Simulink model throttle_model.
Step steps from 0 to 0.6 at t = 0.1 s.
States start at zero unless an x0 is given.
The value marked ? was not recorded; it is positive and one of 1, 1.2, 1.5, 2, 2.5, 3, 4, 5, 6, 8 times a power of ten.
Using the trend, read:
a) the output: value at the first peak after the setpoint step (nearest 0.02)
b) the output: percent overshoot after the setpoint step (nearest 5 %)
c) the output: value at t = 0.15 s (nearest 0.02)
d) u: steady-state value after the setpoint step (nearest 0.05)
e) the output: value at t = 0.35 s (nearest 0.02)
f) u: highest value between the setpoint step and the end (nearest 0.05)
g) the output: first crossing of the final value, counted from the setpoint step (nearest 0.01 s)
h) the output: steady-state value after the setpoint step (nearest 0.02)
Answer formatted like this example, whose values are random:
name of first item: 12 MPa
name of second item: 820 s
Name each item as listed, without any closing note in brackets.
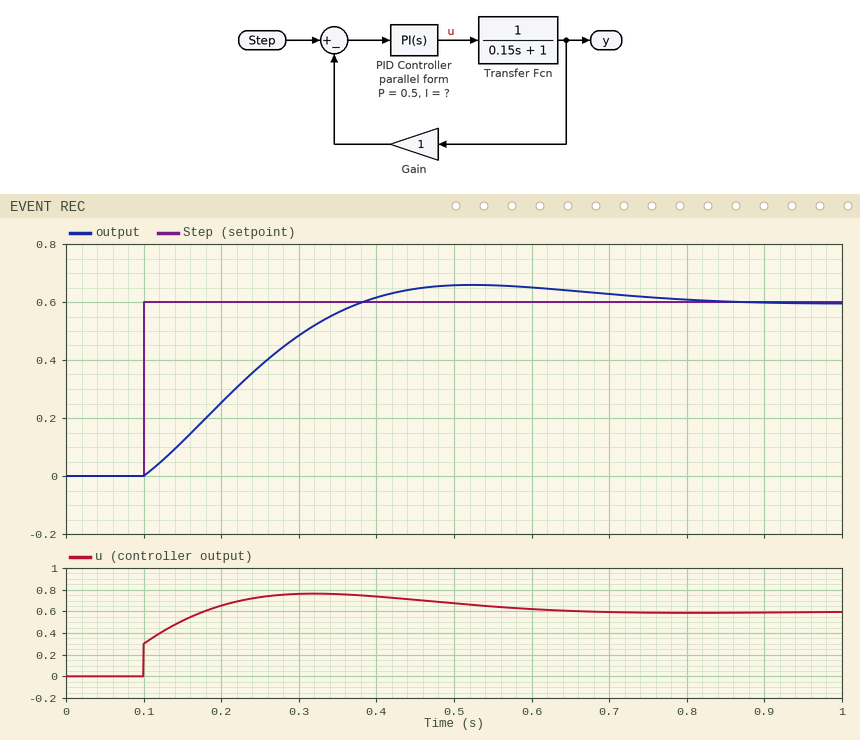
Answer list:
the output: value at the first peak after the setpoint step: 0.66
the output: percent overshoot after the setpoint step: 10 %
the output: value at t = 0.15 s: 0.12
u: steady-state value after the setpoint step: 0.60
the output: value at t = 0.35 s: 0.56
u: highest value between the setpoint step and the end: 0.75
the output: first crossing of the final value, counted from the setpoint step: 0.28 s
the output: steady-state value after the setpoint step: 0.60
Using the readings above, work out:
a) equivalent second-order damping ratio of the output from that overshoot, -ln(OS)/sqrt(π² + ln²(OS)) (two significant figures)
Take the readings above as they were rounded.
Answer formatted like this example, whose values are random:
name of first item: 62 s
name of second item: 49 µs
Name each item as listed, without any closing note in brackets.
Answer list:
equivalent second-order damping ratio of the output from that overshoot, -ln(OS)/sqrt(π² + ln²(OS)): 0.59
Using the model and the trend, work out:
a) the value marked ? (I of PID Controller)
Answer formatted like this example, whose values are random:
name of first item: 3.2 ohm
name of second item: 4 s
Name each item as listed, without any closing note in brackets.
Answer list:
the value marked ?: 10
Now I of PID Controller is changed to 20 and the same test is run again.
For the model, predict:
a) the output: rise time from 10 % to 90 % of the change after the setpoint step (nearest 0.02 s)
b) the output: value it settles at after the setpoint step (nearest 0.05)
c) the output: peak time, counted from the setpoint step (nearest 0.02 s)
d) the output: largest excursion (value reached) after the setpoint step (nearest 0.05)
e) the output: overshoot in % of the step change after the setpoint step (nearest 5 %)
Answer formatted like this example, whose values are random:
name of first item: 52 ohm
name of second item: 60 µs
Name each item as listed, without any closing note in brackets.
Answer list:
the output: rise time from 10 % to 90 % of the change after the setpoint step: 0.12 s
the output: value it settles at after the setpoint step: 0.60
the output: peak time, counted from the setpoint step: 0.28 s
the output: largest excursion (value reached) after the setpoint step: 0.75
the output: overshoot in % of the step change after the setpoint step: 25 %
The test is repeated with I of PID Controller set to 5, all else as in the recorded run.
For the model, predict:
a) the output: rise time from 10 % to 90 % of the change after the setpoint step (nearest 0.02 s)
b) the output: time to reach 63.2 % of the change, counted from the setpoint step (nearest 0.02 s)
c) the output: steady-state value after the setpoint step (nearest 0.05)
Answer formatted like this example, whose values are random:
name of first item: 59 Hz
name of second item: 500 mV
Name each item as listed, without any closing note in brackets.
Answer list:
the output: rise time from 10 % to 90 % of the change after the setpoint step: 0.40 s
the output: time to reach 63.2 % of the change, counted from the setpoint step: 0.22 s
the output: steady-state value after the setpoint step: 0.60
